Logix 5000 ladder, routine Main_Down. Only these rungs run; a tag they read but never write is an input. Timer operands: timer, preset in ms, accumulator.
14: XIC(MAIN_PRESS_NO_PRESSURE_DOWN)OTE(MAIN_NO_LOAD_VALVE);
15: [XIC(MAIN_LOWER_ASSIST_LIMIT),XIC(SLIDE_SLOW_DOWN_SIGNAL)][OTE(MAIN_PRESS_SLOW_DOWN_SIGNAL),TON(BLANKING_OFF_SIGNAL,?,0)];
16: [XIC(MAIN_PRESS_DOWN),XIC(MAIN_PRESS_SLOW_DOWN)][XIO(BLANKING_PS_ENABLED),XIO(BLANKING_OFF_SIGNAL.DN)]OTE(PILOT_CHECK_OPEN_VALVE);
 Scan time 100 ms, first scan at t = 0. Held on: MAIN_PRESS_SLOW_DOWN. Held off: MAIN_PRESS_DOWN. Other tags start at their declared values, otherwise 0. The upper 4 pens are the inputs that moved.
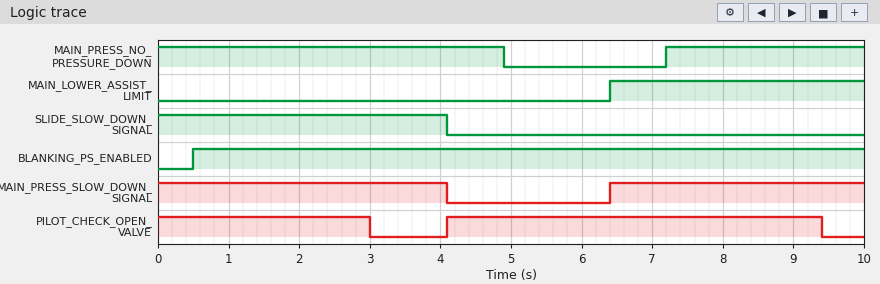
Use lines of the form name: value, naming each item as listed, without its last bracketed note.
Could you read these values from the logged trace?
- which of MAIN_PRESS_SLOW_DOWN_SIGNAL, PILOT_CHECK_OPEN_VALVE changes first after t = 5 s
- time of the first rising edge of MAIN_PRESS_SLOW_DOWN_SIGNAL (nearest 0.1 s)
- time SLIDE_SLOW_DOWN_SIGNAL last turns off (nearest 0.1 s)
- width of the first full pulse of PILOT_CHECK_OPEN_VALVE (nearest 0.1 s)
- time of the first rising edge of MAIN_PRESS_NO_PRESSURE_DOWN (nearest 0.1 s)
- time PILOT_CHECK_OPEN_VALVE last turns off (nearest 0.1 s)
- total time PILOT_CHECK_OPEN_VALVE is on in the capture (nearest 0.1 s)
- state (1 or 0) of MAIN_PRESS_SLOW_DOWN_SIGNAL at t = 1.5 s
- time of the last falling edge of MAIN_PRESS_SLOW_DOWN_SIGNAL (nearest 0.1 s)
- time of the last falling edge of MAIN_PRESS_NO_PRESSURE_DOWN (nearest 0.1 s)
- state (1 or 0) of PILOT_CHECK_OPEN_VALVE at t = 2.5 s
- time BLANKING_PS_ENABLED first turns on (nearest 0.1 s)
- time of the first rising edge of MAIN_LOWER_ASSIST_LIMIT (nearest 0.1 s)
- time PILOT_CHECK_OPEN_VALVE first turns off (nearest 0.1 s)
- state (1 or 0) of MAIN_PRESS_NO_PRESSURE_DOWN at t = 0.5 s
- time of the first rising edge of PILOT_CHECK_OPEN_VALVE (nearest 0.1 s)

which of MAIN_PRESS_SLOW_DOWN_SIGNAL, PILOT_CHECK_OPEN_VALVE changes first after t = 5 s: MAIN_PRESS_SLOW_DOWN_SIGNAL
time of the first rising edge of MAIN_PRESS_SLOW_DOWN_SIGNAL: 6.4 s
time SLIDE_SLOW_DOWN_SIGNAL last turns off: 4.1 s
width of the first full pulse of PILOT_CHECK_OPEN_VALVE: 5.3 s
time of the first rising edge of MAIN_PRESS_NO_PRESSURE_DOWN: 7.2 s
time PILOT_CHECK_OPEN_VALVE last turns off: 9.4 s
total time PILOT_CHECK_OPEN_VALVE is on in the capture: 8.3 s
state (1 or 0) of MAIN_PRESS_SLOW_DOWN_SIGNAL at t = 1.5 s: 1
time of the last falling edge of MAIN_PRESS_SLOW_DOWN_SIGNAL: 4.1 s
time of the last falling edge of MAIN_PRESS_NO_PRESSURE_DOWN: 4.9 s
state (1 or 0) of PILOT_CHECK_OPEN_VALVE at t = 2.5 s: 1
time BLANKING_PS_ENABLED first turns on: 0.5 s
time of the first rising edge of MAIN_LOWER_ASSIST_LIMIT: 6.4 s
time PILOT_CHECK_OPEN_VALVE first turns off: 3.0 s
state (1 or 0) of MAIN_PRESS_NO_PRESSURE_DOWN at t = 0.5 s: 1
time of the first rising edge of PILOT_CHECK_OPEN_VALVE: 4.1 s
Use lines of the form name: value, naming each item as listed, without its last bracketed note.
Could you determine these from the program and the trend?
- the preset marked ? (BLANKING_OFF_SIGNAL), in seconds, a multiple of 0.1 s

the preset marked ? (BLANKING_OFF_SIGNAL), in seconds, a multiple of 0.1 s: 3.0 s
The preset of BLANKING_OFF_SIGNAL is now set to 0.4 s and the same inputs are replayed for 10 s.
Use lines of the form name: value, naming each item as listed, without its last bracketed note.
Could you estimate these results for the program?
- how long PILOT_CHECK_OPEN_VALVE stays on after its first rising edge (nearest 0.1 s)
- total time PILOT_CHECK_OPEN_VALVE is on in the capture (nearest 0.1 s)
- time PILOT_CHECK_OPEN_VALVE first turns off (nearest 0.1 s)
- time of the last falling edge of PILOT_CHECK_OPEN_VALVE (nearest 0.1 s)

how long PILOT_CHECK_OPEN_VALVE stays on after its first rising edge: 2.7 s
total time PILOT_CHECK_OPEN_VALVE is on in the capture: 3.2 s
time PILOT_CHECK_OPEN_VALVE first turns off: 0.5 s
time of the last falling edge of PILOT_CHECK_OPEN_VALVE: 6.8 s
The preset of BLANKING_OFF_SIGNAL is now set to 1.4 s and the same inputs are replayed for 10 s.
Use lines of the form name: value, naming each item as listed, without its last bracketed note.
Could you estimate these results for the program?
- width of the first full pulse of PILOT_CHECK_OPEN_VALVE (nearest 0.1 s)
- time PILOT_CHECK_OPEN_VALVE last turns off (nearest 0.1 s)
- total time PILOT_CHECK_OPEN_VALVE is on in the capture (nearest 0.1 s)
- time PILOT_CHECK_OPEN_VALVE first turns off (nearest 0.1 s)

width of the first full pulse of PILOT_CHECK_OPEN_VALVE: 3.7 s
time PILOT_CHECK_OPEN_VALVE last turns off: 7.8 s
total time PILOT_CHECK_OPEN_VALVE is on in the capture: 5.1 s
time PILOT_CHECK_OPEN_VALVE first turns off: 1.4 s
